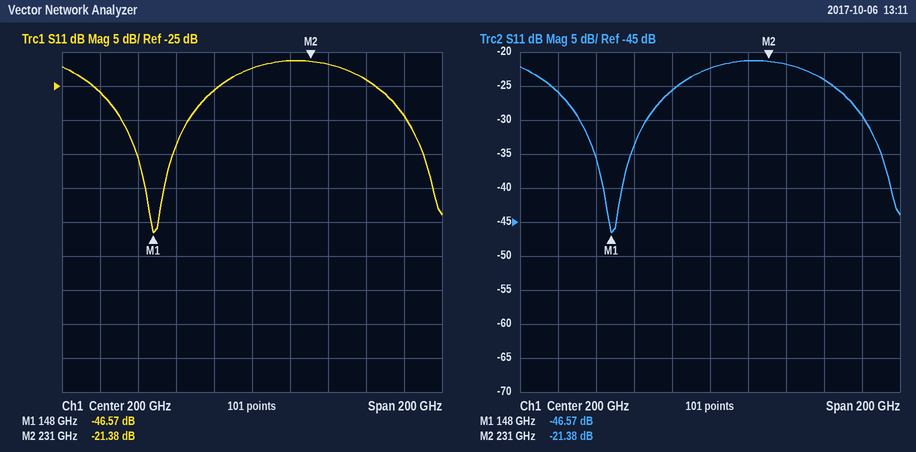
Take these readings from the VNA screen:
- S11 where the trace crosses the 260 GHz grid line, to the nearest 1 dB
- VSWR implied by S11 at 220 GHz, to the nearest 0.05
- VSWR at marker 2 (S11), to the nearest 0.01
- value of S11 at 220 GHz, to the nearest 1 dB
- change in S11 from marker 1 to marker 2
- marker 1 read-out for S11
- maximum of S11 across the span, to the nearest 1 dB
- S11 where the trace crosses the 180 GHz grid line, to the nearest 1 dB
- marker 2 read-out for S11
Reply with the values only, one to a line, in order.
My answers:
-24 dB
1.20
1.19
-21 dB
25.19 dB
-46.57 dB
-21 dB
-26 dB
-21.38 dB
